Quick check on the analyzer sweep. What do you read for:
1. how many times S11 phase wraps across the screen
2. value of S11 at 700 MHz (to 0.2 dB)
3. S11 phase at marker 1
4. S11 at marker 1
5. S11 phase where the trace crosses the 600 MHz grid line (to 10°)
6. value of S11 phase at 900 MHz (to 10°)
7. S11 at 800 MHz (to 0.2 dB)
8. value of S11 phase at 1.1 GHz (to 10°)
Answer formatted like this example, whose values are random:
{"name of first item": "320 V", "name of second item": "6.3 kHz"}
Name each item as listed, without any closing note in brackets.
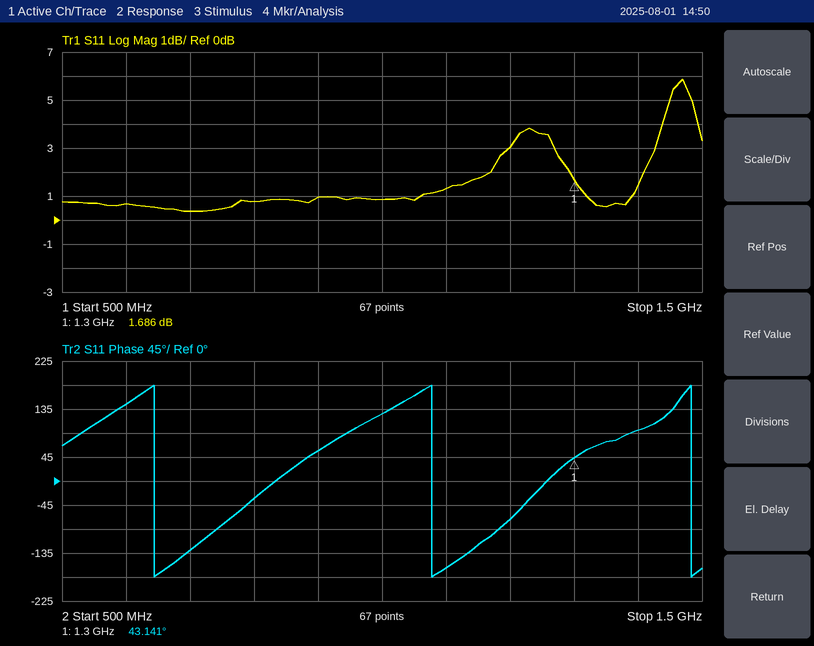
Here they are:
{"how many times S11 phase wraps across the screen": "3", "value of S11 at 700 MHz": "0.4 dB", "S11 phase at marker 1": "43.141°", "S11 at marker 1": "1.686 dB", "S11 phase where the trace crosses the 600 MHz grid line": "140°", "value of S11 phase at 900 MHz": "60°", "S11 at 800 MHz": "0.8 dB", "value of S11 phase at 1.1 GHz": "-160°"}
